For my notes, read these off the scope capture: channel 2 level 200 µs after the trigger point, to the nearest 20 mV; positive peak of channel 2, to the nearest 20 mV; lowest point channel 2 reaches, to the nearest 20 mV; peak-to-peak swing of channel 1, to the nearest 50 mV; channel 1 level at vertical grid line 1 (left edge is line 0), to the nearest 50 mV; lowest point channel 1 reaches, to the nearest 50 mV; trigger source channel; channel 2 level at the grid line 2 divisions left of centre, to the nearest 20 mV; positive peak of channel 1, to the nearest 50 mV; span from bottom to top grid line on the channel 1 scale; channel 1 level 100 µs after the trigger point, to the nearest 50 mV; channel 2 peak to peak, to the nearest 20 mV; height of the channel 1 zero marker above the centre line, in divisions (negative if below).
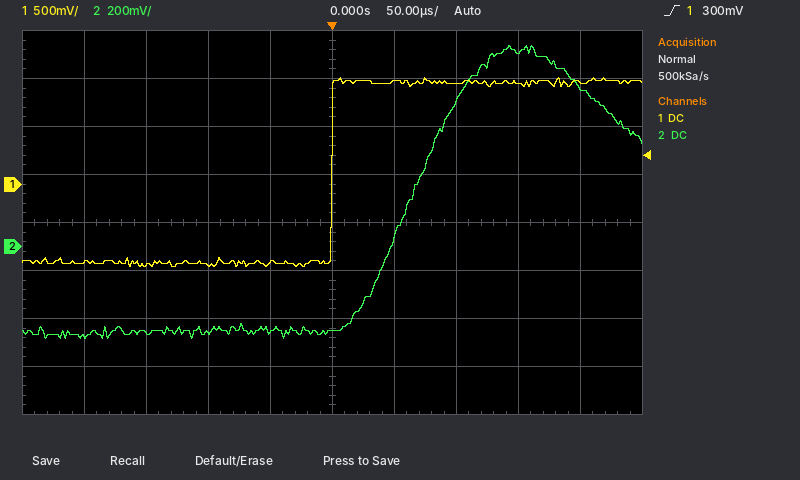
660 mV
840 mV
-380 mV
1.95 V
-800 mV
-850 mV
channel 1
-360 mV
1.10 V
4 V
1.05 V
1.22 V
+0.8 div
